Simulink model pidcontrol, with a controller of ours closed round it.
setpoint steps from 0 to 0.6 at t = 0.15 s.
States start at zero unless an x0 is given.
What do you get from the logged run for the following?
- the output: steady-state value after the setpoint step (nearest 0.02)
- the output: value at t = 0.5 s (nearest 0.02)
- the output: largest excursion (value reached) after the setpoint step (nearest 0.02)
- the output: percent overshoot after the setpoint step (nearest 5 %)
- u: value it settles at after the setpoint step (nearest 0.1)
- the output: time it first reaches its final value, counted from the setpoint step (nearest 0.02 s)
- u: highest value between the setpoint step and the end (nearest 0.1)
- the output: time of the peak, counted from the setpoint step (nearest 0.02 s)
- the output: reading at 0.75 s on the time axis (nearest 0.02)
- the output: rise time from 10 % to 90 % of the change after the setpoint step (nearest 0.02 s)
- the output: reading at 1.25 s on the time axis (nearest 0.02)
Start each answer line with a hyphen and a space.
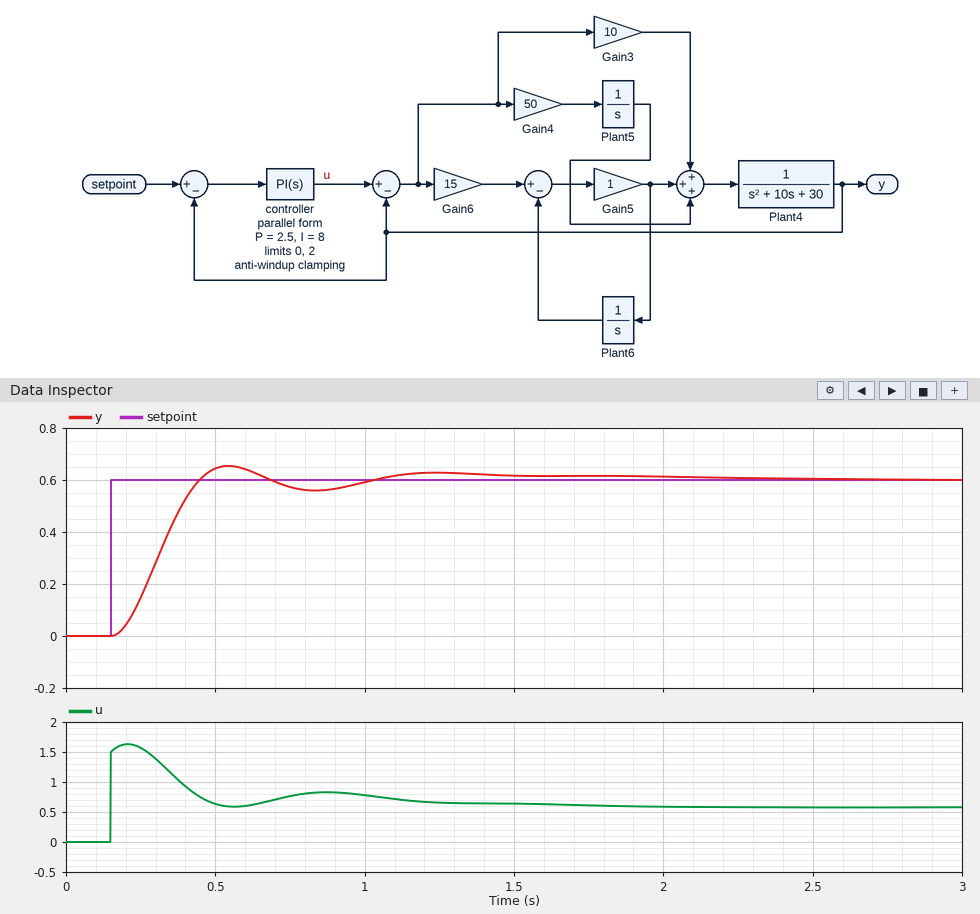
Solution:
- 0.60
- 0.64
- 0.66
- 10 %
- 0.6
- 0.30 s
- 1.6
- 0.40 s
- 0.58
- 0.20 s
- 0.62
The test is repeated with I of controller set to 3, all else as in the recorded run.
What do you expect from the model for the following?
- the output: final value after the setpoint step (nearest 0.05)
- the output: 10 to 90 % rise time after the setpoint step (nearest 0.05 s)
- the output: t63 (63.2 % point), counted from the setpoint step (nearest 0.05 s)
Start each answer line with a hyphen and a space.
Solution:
- 0.60
- 0.90 s
- 0.20 s
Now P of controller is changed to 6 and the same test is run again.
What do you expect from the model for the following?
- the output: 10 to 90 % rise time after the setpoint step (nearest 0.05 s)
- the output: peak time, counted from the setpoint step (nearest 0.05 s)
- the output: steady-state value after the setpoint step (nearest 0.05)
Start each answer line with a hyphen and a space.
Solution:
- 0.15 s
- 0.30 s
- 0.60
